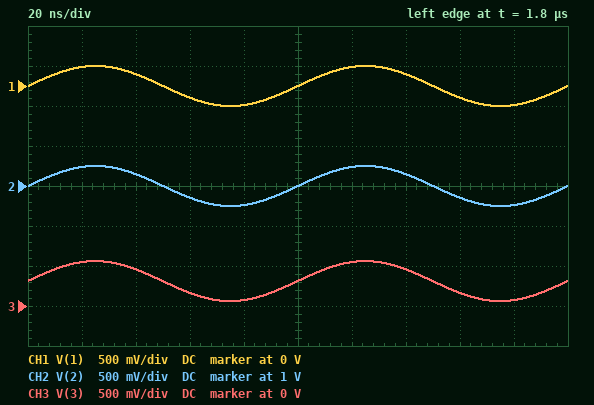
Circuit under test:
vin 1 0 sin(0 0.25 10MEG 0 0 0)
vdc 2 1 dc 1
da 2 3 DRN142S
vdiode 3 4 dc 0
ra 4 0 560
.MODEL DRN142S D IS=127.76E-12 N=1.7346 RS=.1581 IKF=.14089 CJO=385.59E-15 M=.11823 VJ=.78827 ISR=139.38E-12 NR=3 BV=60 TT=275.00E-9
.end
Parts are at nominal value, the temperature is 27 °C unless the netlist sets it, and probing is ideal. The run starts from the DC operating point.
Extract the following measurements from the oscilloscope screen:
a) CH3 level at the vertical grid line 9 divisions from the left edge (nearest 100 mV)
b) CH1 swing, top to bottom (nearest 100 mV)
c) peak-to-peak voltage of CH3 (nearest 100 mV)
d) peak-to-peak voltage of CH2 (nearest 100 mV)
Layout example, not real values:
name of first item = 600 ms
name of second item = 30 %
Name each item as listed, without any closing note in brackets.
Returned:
CH3 level at the vertical grid line 9 divisions from the left edge = 100 mV
CH1 swing, top to bottom = 500 mV
peak-to-peak voltage of CH3 = 500 mV
peak-to-peak voltage of CH2 = 500 mV
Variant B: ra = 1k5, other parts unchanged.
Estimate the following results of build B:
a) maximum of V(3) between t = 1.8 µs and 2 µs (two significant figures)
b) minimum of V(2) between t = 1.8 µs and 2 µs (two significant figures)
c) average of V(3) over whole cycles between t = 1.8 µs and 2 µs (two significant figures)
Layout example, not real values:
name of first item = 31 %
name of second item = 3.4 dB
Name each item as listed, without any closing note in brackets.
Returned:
maximum of V(3) between t = 1.8 µs and 2 µs = 600 mV
minimum of V(2) between t = 1.8 µs and 2 µs = 750 mV
average of V(3) over whole cycles between t = 1.8 µs and 2 µs = 350 mV
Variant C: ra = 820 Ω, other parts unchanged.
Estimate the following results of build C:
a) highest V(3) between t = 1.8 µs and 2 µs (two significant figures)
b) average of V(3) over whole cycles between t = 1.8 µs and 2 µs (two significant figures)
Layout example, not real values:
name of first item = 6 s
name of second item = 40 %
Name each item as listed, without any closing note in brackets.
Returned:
highest V(3) between t = 1.8 µs and 2 µs = 580 mV
average of V(3) over whole cycles between t = 1.8 µs and 2 µs = 330 mV
